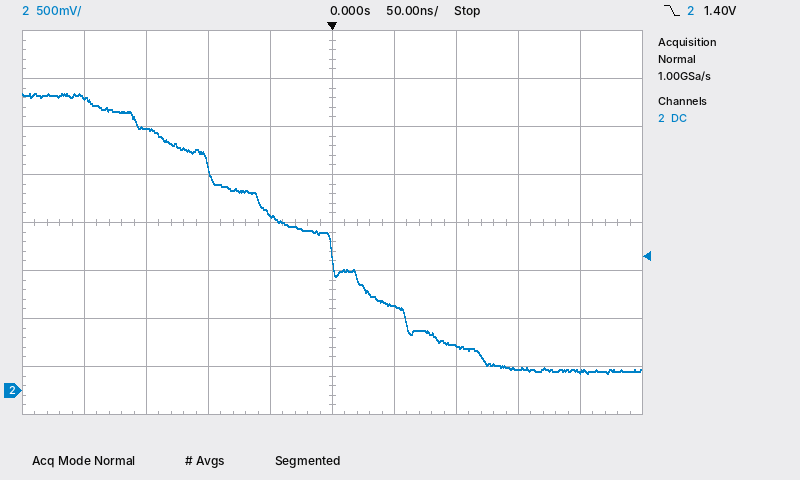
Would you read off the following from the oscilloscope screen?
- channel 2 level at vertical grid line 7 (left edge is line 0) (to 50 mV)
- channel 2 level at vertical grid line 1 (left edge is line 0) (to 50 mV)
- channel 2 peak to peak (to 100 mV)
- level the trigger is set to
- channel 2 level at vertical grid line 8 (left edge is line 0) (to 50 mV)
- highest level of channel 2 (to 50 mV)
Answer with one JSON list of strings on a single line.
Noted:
["450 mV", "3.05 V", "2.90 V", "1.40 V", "200 mV", "3.10 V"]
